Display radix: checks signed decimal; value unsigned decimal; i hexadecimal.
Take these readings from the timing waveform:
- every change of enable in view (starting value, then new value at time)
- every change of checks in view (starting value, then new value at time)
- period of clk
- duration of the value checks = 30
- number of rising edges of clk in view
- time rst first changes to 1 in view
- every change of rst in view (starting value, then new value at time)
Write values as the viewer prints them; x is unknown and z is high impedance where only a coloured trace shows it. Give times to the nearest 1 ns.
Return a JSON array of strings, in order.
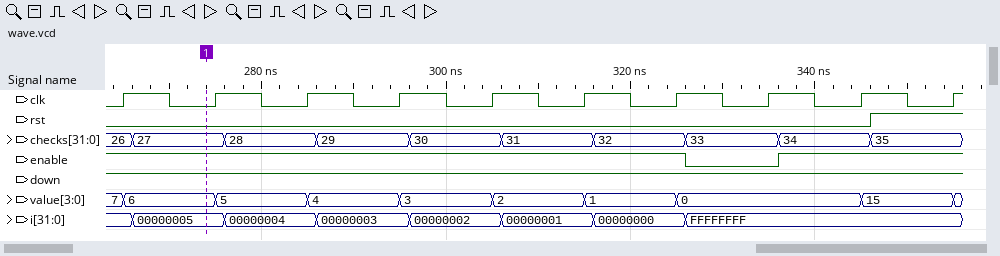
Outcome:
["1, 0 at 326 ns, 1 at 336 ns", "26, 27 at 266 ns, 28 at 276 ns, 29 at 286 ns, 30 at 296 ns, 31 at 306 ns, 32 at 316 ns, 33 at 326 ns, 34 at 336 ns, 35 at 346 ns", "10 ns", "10 ns", "10", "346 ns", "0, 1 at 346 ns"]
